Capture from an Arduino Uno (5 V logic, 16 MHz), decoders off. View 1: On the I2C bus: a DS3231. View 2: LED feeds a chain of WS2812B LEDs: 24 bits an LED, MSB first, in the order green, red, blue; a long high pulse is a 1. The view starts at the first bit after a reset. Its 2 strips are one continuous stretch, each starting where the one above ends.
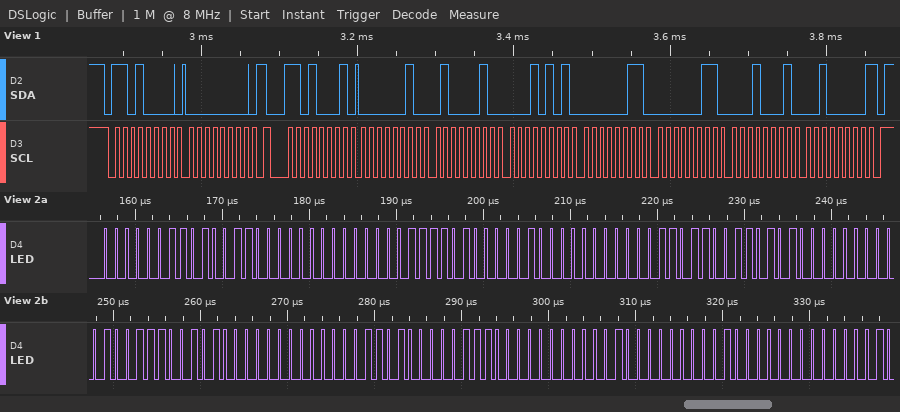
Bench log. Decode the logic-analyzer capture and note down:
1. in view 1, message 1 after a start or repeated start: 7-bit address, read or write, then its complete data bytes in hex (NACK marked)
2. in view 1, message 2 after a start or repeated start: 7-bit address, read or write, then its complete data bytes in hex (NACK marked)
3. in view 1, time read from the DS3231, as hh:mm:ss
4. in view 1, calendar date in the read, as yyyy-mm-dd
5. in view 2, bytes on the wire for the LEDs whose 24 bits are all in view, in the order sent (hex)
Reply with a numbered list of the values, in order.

1. 0x68 write: 00
2. 0x68 read: 02 42 15 03 03 11 20 NACK
3. 15:42:02
4. 2020-11-03
5. 03 4C 00 0F 41 00 1B 35 00 27 28 00 34 1C 00 40 10 00
